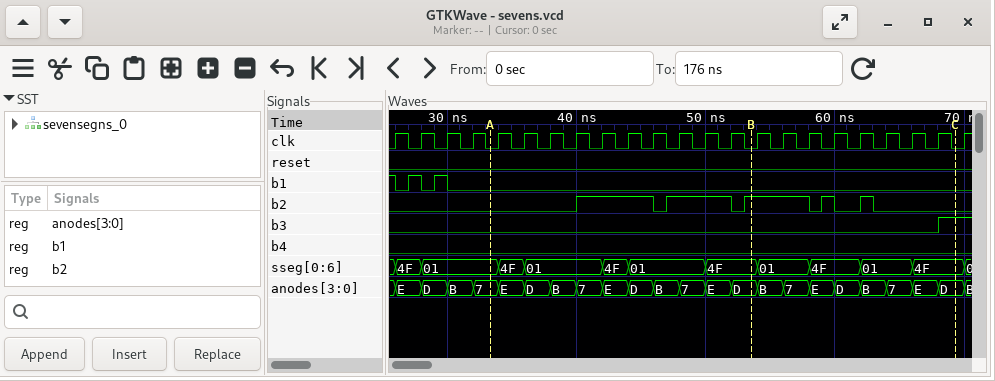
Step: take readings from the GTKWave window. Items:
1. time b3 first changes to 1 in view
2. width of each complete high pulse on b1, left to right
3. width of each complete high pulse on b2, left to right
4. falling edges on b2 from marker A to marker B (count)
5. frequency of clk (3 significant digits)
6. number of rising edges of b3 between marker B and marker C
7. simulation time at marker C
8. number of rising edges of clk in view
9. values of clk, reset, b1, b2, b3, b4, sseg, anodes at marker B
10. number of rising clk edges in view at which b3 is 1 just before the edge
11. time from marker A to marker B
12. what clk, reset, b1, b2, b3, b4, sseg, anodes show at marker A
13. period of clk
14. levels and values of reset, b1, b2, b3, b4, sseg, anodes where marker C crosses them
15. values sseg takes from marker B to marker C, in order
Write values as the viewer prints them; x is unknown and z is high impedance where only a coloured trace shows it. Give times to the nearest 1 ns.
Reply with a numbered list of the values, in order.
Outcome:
1. 68 ns
2. 1 ns, 1 ns
3. 6 ns, 5 ns, 5 ns, 1 ns, 1 ns
4. 2
5. 500 MHz
6. 1
7. 69 ns
8. 23
9. clk=0, reset=0, b1=0, b2=1, b3=0, b4=0, sseg=4F, anodes=D
10. 1
11. 20 ns
12. clk=0, reset=0, b1=0, b2=0, b3=0, b4=0, sseg=01, anodes=7
13. 2 ns
14. reset=0, b1=0, b2=0, b3=1, b4=0, sseg=4F, anodes=D
15. 4F, 01, 4F, 01, 4F
